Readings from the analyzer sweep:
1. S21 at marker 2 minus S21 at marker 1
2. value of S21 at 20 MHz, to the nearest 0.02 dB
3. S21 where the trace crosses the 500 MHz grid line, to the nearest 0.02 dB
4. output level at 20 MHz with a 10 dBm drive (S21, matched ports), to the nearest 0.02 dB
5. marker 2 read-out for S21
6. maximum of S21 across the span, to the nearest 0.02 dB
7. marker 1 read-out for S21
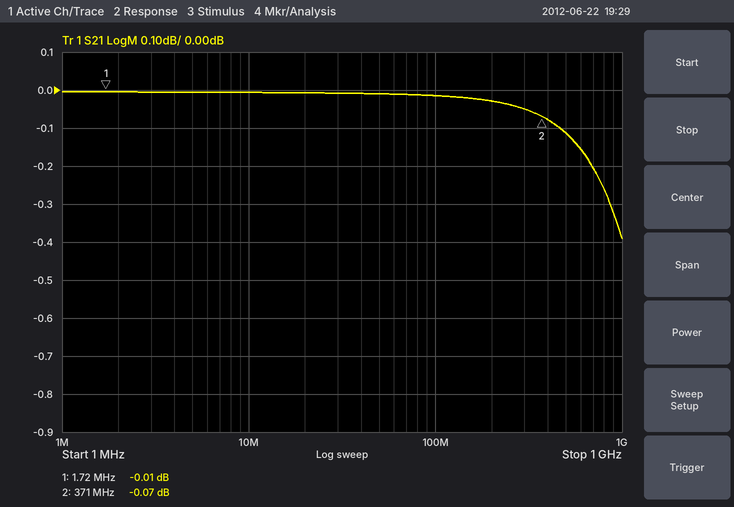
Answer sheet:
-0.06 dB
0.00 dB
-0.12 dB
10.00 dBm
-0.07 dB
0.00 dB
-0.01 dB
